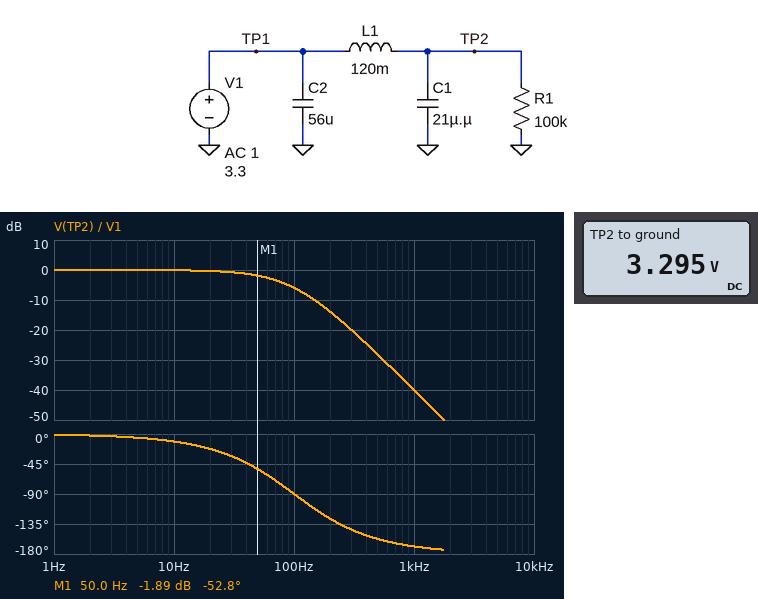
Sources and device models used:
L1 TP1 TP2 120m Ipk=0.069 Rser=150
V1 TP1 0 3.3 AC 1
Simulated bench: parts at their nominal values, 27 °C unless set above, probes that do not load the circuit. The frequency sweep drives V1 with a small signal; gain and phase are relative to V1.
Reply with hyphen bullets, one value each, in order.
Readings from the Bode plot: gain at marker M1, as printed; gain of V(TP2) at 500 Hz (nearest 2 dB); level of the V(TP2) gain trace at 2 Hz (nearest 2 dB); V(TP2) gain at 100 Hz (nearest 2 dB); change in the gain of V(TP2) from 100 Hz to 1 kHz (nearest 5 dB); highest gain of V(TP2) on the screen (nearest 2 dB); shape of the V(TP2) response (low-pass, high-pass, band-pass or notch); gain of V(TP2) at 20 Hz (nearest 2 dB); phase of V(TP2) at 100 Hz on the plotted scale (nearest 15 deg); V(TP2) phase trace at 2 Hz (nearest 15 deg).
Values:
- -1.89 dB
- -28 dB
- 0 dB
- -6 dB
- -35 dB
- 0 dB
- low-pass
- 0 dB
- -90 deg
- 0 deg
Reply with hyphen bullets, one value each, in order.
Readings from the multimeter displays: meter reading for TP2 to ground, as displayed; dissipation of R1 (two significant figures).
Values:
- 3.295 V
- 110 µW
